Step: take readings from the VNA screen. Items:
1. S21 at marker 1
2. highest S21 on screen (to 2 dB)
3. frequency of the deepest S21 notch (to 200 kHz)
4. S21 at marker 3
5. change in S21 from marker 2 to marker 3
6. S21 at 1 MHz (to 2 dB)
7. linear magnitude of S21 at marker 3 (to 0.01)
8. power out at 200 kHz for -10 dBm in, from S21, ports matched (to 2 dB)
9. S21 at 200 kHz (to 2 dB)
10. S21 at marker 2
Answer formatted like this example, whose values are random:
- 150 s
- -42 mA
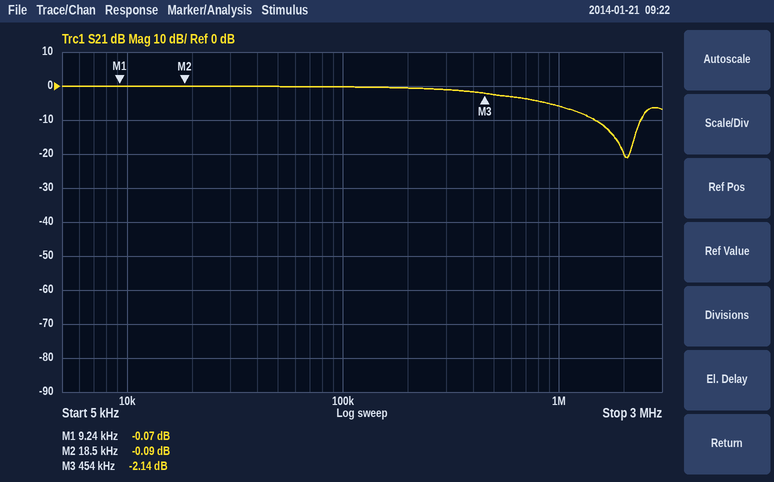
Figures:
- -0.07 dB
- 0 dB
- 2.0 MHz
- -2.14 dB
- -2.05 dB
- -6 dB
- 0.78
- -10 dBm
- 0 dB
- -0.09 dB
